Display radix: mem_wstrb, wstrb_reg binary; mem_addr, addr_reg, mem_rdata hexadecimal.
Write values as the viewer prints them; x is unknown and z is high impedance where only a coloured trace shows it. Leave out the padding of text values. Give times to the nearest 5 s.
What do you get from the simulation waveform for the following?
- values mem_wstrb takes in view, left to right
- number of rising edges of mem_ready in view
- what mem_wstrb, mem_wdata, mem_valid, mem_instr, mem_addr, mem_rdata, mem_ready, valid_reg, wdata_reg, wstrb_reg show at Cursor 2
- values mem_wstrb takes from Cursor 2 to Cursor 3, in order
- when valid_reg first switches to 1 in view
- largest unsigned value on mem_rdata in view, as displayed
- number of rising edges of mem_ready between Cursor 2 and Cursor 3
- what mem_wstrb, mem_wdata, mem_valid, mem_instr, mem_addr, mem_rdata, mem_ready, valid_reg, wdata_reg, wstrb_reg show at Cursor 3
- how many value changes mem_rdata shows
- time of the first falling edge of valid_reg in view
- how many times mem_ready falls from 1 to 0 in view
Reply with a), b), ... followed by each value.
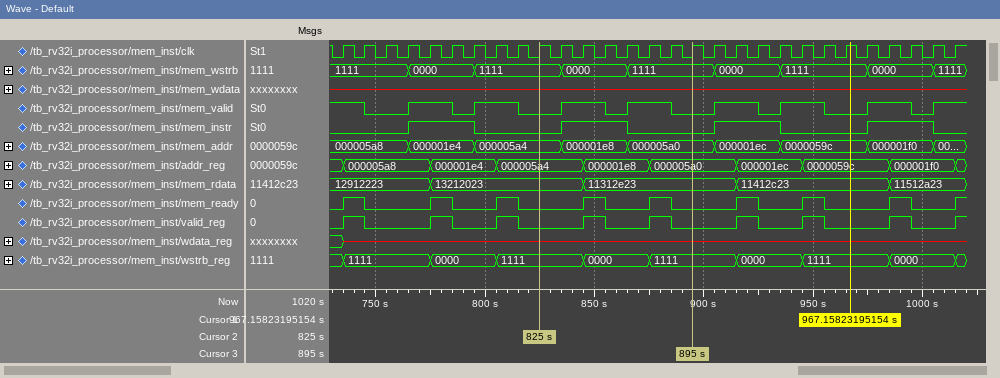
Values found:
a) 1111, 0000, 1111, 0000, 1111, 0000, 1111, 0000, 1111
b) 9
c) mem_wstrb=1111, mem_wdata=x, mem_valid=0, mem_instr=0, mem_addr=000005a4, mem_rdata=13212023, mem_ready=0, valid_reg=0, wdata_reg=x, wstrb_reg=1111
d) 1111, 0000, 1111
e) 735 s
f) 13212023
g) 2
h) mem_wstrb=1111, mem_wdata=x, mem_valid=0, mem_instr=0, mem_addr=000005a0, mem_rdata=11312e23, mem_ready=0, valid_reg=0, wdata_reg=x, wstrb_reg=1111
i) 4
j) 745 s
k) 8
